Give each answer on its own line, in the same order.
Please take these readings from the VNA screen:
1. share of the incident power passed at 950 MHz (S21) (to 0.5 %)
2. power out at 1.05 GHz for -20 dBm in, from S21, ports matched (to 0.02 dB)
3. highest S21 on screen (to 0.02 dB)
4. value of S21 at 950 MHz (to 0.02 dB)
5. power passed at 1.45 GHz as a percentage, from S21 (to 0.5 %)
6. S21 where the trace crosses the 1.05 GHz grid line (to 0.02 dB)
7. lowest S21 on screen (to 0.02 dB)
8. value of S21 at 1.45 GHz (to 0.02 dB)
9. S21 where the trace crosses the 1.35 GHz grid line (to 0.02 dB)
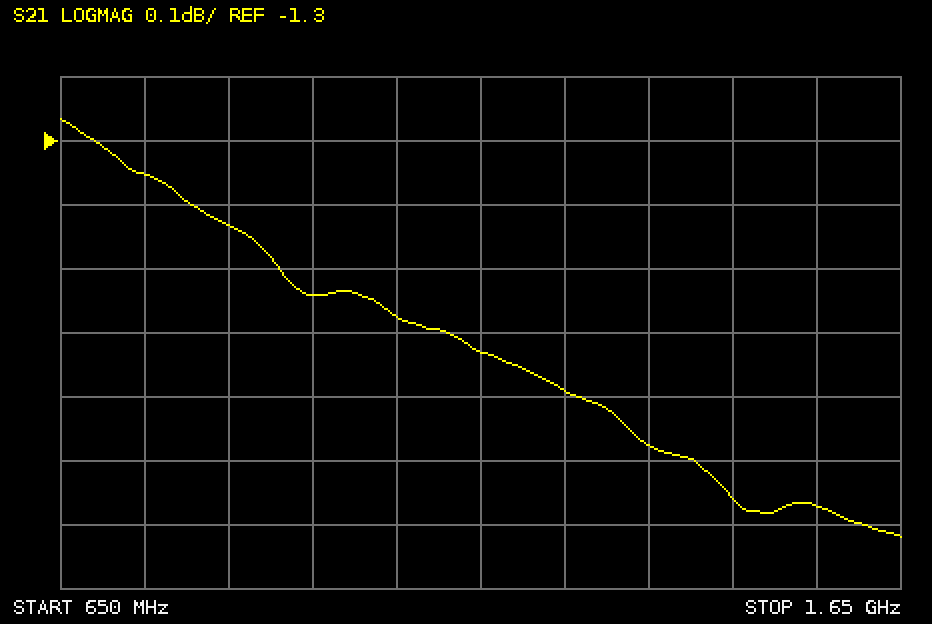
70.0 %
-21.58 dBm
-1.26 dB
-1.54 dB
65.0 %
-1.58 dB
-1.92 dB
-1.86 dB
-1.78 dB
